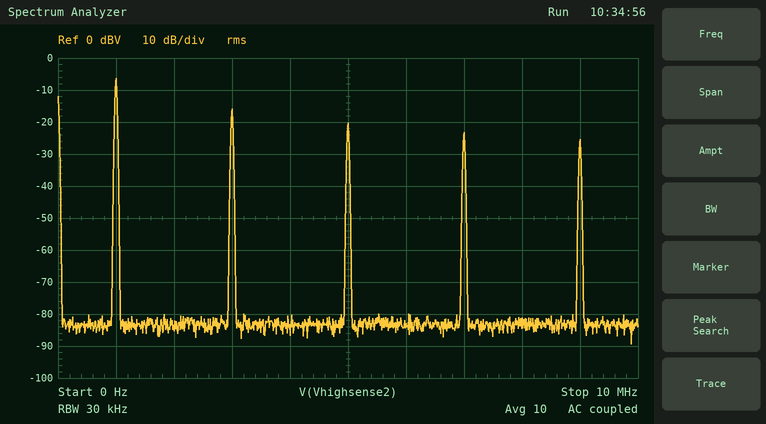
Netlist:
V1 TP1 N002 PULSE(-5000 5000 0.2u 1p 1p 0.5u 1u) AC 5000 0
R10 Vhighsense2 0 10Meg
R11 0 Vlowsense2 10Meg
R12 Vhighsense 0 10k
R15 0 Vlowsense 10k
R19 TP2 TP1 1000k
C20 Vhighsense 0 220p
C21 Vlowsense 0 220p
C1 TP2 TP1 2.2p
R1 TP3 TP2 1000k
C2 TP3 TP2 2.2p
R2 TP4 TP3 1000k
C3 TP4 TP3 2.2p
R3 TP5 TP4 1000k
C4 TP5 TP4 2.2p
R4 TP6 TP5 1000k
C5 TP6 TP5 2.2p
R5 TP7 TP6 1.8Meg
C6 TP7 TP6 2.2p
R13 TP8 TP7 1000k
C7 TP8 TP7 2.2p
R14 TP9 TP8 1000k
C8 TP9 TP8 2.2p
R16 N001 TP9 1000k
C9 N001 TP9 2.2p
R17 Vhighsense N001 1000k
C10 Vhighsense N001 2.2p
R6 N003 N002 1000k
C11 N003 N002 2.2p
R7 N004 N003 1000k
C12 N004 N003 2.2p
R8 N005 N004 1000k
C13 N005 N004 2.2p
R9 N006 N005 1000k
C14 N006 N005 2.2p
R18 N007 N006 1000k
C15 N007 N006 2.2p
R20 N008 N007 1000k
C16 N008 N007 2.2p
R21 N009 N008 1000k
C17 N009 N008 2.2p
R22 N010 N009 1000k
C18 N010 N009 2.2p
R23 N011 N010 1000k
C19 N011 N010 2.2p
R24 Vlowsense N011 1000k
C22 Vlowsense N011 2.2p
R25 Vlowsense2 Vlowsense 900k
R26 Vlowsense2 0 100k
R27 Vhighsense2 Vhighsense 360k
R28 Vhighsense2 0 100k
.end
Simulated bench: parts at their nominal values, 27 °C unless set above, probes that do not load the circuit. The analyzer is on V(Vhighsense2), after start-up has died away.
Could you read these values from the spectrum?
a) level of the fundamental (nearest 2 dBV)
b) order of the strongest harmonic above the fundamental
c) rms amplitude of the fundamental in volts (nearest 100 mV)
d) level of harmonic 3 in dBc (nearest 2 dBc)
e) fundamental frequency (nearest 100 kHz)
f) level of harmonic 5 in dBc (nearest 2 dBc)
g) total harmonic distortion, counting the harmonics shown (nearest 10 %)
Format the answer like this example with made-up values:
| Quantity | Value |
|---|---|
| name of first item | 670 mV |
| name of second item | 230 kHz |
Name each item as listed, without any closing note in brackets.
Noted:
| Quantity | Value |
|---|---|
| level of the fundamental | -6 dBV |
| order of the strongest harmonic above the fundamental | 3 |
| rms amplitude of the fundamental in volts | 500 mV |
| level of harmonic 3 in dBc | -10 dBc |
| fundamental frequency | 1.0 MHz |
| level of harmonic 5 in dBc | -14 dBc |
| total harmonic distortion, counting the harmonics shown | 40 % |
